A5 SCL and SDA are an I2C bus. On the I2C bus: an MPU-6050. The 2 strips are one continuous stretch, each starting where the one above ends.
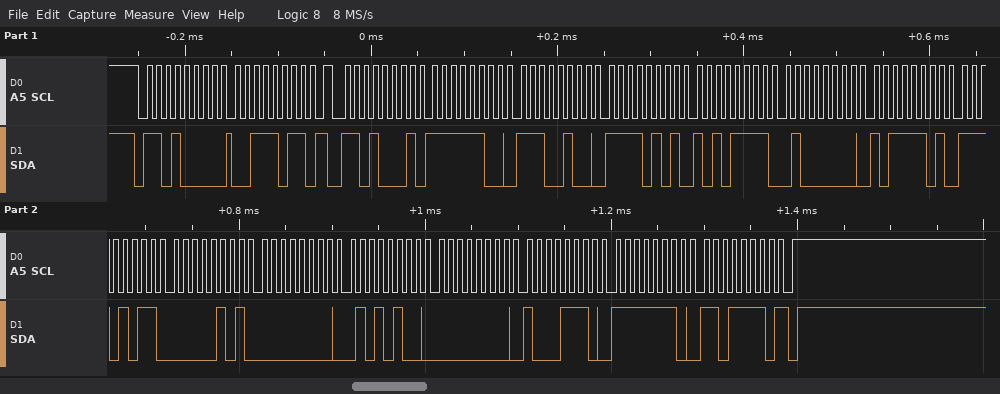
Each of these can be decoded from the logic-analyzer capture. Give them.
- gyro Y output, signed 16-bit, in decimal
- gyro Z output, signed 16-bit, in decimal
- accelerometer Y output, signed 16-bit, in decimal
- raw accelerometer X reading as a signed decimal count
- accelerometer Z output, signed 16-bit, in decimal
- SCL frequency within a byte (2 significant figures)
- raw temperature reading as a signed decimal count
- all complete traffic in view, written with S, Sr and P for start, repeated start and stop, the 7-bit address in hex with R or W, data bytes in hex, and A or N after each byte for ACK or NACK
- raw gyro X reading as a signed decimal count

142
-290
-2641
-796
16573
100 kHz
-5371
S 68W A 3B A Sr 68R A FC A E4 A F5 A AF A 40 A BD A EB A 05 A 00 A 54 A 00 A 8E A FE A DE N P
84
